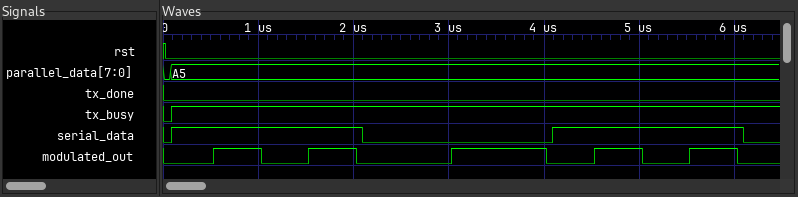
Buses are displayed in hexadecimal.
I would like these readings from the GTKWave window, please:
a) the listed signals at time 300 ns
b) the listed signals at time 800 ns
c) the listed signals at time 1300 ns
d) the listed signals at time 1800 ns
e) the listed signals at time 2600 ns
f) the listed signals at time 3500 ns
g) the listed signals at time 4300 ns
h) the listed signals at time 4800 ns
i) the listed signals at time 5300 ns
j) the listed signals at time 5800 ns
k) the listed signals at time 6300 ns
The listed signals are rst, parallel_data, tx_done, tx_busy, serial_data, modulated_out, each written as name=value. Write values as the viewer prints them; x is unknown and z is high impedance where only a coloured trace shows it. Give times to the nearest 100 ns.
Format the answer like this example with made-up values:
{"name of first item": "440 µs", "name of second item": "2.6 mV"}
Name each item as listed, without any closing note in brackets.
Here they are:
{"the listed signals at time 300 ns": "rst=0, parallel_data=A5, tx_done=0, tx_busy=1, serial_data=1, modulated_out=0", "the listed signals at time 800 ns": "rst=0, parallel_data=A5, tx_done=0, tx_busy=1, serial_data=1, modulated_out=1", "the listed signals at time 1300 ns": "rst=0, parallel_data=A5, tx_done=0, tx_busy=1, serial_data=1, modulated_out=0", "the listed signals at time 1800 ns": "rst=0, parallel_data=A5, tx_done=0, tx_busy=1, serial_data=1, modulated_out=1", "the listed signals at time 2600 ns": "rst=0, parallel_data=A5, tx_done=0, tx_busy=1, serial_data=0, modulated_out=0", "the listed signals at time 3500 ns": "rst=0, parallel_data=A5, tx_done=0, tx_busy=1, serial_data=0, modulated_out=1", "the listed signals at time 4300 ns": "rst=0, parallel_data=A5, tx_done=0, tx_busy=1, serial_data=1, modulated_out=0", "the listed signals at time 4800 ns": "rst=0, parallel_data=A5, tx_done=0, tx_busy=1, serial_data=1, modulated_out=1", "the listed signals at time 5300 ns": "rst=0, parallel_data=A5, tx_done=0, tx_busy=1, serial_data=1, modulated_out=0", "the listed signals at time 5800 ns": "rst=0, parallel_data=A5, tx_done=0, tx_busy=1, serial_data=1, modulated_out=1", "the listed signals at time 6300 ns": "rst=0, parallel_data=A5, tx_done=0, tx_busy=1, serial_data=0, modulated_out=0"}
